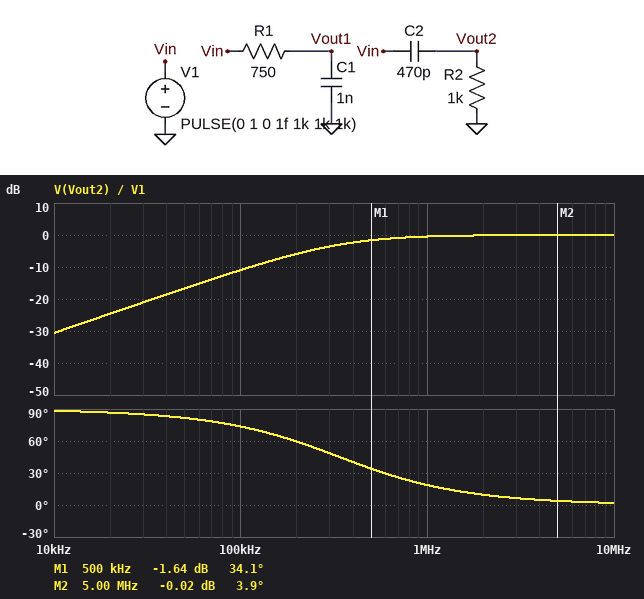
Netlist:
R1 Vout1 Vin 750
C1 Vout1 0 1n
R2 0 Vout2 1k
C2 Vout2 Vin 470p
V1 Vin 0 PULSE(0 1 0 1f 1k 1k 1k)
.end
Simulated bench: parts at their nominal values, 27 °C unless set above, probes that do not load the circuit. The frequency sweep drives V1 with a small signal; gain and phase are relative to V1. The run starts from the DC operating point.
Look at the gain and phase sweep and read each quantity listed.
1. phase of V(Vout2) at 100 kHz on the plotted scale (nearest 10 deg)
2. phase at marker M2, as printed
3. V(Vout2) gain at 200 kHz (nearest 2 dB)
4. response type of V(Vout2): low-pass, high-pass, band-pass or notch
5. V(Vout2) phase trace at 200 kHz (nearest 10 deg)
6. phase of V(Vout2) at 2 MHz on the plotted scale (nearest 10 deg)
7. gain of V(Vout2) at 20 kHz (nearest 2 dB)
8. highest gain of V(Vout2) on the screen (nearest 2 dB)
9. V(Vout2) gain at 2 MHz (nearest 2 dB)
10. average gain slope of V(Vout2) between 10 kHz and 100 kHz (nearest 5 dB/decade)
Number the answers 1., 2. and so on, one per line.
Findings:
1. 70 deg
2. 3.9 deg
3. -6 dB
4. high-pass
5. 60 deg
6. 10 deg
7. -24 dB
8. 0 dB
9. 0 dB
10. 20 dB/decade
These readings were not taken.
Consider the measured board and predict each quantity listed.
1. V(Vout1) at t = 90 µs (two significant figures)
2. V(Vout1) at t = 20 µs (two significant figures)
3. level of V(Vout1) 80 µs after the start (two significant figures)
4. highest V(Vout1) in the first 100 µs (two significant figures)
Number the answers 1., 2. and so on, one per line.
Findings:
1. 1.0 V
2. 1.0 V
3. 1.0 V
4. 1.0 V
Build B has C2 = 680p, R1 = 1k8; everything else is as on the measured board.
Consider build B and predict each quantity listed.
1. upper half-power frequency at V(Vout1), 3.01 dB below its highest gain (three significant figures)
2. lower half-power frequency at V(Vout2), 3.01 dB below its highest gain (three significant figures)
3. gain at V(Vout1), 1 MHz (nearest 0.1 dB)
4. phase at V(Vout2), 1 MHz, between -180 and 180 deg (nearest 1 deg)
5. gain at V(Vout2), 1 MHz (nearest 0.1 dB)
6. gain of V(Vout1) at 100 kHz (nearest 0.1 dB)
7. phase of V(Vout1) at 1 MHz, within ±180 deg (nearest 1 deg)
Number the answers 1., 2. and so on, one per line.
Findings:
1. 88.4 kHz
2. 234 kHz
3. -21.1 dB
4. 13 deg
5. -0.2 dB
6. -3.6 dB
7. -85 deg
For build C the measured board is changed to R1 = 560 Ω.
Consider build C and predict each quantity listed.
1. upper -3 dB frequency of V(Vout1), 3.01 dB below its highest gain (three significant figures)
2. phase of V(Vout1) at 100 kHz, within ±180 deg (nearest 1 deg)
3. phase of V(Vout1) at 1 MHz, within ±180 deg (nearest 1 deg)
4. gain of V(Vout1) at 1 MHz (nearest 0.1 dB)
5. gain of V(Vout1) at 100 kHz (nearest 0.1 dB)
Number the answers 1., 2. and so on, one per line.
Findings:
1. 284 kHz
2. -19 deg
3. -74 deg
4. -11.3 dB
5. -0.5 dB
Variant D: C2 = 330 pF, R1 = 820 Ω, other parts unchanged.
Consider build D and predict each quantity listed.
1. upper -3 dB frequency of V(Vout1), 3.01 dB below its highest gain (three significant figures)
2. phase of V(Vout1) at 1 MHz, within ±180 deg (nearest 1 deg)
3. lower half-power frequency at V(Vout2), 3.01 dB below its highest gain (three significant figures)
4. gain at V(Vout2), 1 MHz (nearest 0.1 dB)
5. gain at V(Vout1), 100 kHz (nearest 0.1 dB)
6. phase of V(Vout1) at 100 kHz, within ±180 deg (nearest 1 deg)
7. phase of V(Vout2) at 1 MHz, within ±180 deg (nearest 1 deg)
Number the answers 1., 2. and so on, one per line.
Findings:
1. 194 kHz
2. -79 deg
3. 482 kHz
4. -0.9 dB
5. -1.0 dB
6. -27 deg
7. 26 deg
